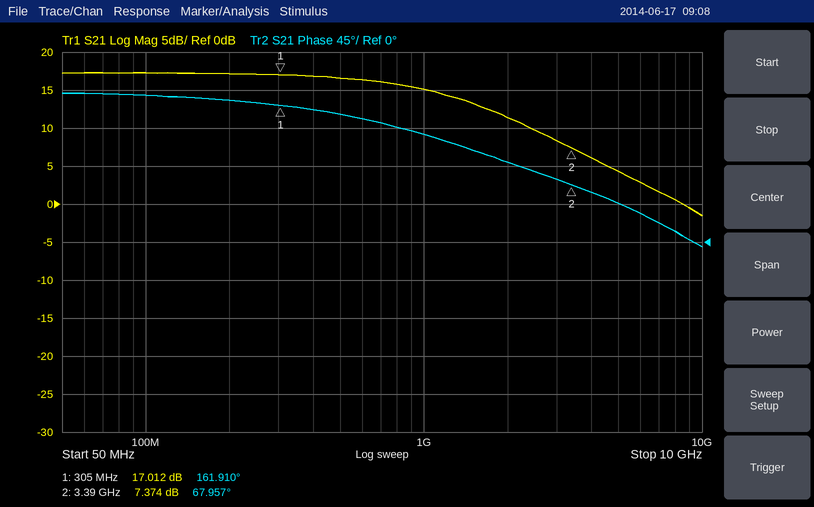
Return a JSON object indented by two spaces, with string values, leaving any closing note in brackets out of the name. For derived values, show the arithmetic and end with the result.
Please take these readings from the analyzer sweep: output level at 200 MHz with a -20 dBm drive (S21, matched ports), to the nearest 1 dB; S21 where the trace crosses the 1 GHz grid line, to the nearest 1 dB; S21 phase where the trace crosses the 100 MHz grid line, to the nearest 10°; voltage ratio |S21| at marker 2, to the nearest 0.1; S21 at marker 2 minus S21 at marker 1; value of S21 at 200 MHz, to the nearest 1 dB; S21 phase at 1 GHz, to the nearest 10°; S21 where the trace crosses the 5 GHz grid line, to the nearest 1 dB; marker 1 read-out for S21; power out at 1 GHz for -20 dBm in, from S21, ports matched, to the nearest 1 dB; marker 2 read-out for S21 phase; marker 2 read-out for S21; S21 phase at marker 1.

{
  "output level at 200 MHz with a -20 dBm drive (S21, matched ports), to the nearest 1 dB": "-20 dBm + (17 dB) = -3 dBm",
  "S21 where the trace crosses the 1 GHz grid line, to the nearest 1 dB": "15 dB",
  "S21 phase where the trace crosses the 100 MHz grid line, to the nearest 10°": "170°",
  "voltage ratio |S21| at marker 2, to the nearest 0.1": "10^(7.374/20) ≈ 2.3",
  "S21 at marker 2 minus S21 at marker 1": "7.374 − (17.012) = -9.638 dB",
  "value of S21 at 200 MHz, to the nearest 1 dB": "17 dB",
  "S21 phase at 1 GHz, to the nearest 10°": "130°",
  "S21 where the trace crosses the 5 GHz grid line, to the nearest 1 dB": "4 dB",
  "marker 1 read-out for S21": "17.012 dB",
  "power out at 1 GHz for -20 dBm in, from S21, ports matched, to the nearest 1 dB": "-20 dBm + (15 dB) = -5 dBm",
  "marker 2 read-out for S21 phase": "67.957°",
  "marker 2 read-out for S21": "7.374 dB",
  "S21 phase at marker 1": "161.910°"
}
